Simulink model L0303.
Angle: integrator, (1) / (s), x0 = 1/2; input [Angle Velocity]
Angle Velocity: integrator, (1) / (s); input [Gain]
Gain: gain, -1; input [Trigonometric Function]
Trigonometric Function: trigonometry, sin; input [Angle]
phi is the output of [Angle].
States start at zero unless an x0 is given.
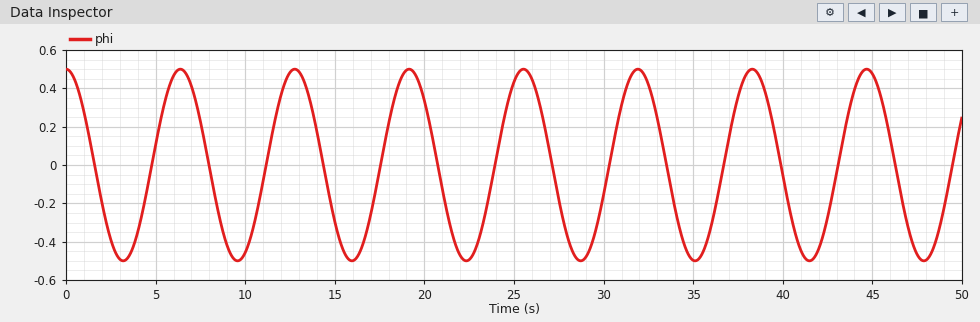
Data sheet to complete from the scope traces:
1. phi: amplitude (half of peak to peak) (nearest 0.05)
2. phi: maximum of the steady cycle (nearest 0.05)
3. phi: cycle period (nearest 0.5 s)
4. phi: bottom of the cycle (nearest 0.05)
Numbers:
0.50
0.50
6.5 s
-0.50
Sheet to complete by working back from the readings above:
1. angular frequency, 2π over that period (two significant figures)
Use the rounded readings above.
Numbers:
0.97 rad/s
